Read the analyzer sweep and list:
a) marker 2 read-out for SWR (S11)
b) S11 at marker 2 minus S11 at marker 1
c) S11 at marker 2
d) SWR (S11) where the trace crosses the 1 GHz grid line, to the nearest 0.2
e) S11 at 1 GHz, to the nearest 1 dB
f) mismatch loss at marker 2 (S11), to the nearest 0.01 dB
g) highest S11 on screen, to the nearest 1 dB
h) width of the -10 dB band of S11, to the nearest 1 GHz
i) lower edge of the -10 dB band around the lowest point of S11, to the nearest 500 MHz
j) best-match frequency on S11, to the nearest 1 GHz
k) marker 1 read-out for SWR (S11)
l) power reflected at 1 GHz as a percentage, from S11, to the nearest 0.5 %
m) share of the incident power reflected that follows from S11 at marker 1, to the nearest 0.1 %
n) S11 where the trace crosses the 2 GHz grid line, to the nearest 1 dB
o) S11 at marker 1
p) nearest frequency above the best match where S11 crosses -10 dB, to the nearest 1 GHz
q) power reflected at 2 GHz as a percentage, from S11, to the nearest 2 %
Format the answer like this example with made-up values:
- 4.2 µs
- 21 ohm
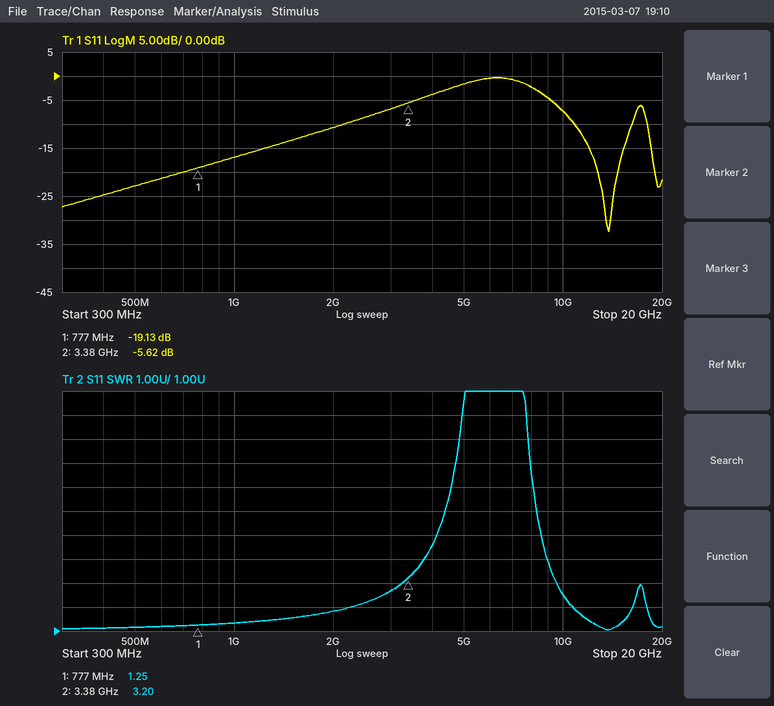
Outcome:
- 3.20
- 13.51 dB
- -5.62 dB
- 1.4
- -17 dB
- 1.39 dB
- 0 dB
- 5 GHz
- 11.0 GHz
- 14 GHz
- 1.25
- 2.0 %
- 1.2 %
- -11 dB
- -19.13 dB
- 16 GHz
- 8 %
